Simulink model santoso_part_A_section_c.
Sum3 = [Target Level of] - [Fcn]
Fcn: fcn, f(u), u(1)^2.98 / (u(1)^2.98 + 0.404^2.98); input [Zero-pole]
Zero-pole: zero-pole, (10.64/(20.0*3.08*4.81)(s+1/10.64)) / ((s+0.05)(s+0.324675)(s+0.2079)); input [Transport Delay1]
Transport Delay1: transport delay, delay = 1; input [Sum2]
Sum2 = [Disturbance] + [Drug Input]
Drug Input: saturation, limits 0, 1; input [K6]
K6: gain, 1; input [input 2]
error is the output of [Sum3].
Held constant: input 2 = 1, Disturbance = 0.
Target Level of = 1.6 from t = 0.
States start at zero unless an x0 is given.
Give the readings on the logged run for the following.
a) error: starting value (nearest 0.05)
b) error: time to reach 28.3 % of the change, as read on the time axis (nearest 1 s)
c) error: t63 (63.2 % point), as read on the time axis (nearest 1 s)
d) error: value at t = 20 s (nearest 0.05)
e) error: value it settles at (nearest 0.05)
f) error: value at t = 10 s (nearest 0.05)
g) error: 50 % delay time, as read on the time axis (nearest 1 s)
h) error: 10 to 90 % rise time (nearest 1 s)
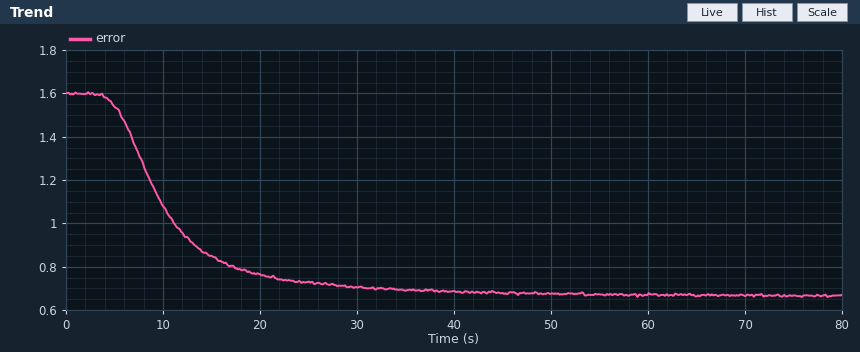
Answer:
1.60
7 s
11 s
0.75
0.65
1.10
9 s
15 s
